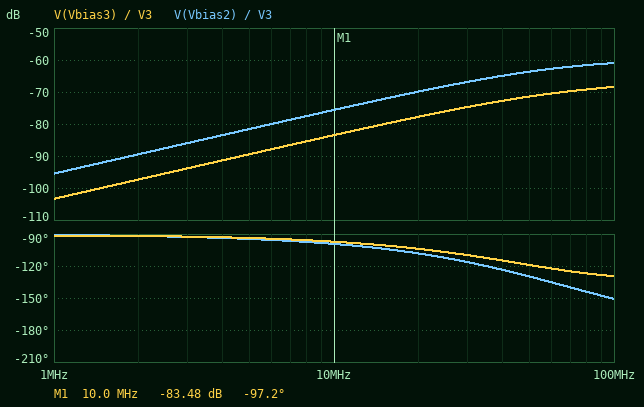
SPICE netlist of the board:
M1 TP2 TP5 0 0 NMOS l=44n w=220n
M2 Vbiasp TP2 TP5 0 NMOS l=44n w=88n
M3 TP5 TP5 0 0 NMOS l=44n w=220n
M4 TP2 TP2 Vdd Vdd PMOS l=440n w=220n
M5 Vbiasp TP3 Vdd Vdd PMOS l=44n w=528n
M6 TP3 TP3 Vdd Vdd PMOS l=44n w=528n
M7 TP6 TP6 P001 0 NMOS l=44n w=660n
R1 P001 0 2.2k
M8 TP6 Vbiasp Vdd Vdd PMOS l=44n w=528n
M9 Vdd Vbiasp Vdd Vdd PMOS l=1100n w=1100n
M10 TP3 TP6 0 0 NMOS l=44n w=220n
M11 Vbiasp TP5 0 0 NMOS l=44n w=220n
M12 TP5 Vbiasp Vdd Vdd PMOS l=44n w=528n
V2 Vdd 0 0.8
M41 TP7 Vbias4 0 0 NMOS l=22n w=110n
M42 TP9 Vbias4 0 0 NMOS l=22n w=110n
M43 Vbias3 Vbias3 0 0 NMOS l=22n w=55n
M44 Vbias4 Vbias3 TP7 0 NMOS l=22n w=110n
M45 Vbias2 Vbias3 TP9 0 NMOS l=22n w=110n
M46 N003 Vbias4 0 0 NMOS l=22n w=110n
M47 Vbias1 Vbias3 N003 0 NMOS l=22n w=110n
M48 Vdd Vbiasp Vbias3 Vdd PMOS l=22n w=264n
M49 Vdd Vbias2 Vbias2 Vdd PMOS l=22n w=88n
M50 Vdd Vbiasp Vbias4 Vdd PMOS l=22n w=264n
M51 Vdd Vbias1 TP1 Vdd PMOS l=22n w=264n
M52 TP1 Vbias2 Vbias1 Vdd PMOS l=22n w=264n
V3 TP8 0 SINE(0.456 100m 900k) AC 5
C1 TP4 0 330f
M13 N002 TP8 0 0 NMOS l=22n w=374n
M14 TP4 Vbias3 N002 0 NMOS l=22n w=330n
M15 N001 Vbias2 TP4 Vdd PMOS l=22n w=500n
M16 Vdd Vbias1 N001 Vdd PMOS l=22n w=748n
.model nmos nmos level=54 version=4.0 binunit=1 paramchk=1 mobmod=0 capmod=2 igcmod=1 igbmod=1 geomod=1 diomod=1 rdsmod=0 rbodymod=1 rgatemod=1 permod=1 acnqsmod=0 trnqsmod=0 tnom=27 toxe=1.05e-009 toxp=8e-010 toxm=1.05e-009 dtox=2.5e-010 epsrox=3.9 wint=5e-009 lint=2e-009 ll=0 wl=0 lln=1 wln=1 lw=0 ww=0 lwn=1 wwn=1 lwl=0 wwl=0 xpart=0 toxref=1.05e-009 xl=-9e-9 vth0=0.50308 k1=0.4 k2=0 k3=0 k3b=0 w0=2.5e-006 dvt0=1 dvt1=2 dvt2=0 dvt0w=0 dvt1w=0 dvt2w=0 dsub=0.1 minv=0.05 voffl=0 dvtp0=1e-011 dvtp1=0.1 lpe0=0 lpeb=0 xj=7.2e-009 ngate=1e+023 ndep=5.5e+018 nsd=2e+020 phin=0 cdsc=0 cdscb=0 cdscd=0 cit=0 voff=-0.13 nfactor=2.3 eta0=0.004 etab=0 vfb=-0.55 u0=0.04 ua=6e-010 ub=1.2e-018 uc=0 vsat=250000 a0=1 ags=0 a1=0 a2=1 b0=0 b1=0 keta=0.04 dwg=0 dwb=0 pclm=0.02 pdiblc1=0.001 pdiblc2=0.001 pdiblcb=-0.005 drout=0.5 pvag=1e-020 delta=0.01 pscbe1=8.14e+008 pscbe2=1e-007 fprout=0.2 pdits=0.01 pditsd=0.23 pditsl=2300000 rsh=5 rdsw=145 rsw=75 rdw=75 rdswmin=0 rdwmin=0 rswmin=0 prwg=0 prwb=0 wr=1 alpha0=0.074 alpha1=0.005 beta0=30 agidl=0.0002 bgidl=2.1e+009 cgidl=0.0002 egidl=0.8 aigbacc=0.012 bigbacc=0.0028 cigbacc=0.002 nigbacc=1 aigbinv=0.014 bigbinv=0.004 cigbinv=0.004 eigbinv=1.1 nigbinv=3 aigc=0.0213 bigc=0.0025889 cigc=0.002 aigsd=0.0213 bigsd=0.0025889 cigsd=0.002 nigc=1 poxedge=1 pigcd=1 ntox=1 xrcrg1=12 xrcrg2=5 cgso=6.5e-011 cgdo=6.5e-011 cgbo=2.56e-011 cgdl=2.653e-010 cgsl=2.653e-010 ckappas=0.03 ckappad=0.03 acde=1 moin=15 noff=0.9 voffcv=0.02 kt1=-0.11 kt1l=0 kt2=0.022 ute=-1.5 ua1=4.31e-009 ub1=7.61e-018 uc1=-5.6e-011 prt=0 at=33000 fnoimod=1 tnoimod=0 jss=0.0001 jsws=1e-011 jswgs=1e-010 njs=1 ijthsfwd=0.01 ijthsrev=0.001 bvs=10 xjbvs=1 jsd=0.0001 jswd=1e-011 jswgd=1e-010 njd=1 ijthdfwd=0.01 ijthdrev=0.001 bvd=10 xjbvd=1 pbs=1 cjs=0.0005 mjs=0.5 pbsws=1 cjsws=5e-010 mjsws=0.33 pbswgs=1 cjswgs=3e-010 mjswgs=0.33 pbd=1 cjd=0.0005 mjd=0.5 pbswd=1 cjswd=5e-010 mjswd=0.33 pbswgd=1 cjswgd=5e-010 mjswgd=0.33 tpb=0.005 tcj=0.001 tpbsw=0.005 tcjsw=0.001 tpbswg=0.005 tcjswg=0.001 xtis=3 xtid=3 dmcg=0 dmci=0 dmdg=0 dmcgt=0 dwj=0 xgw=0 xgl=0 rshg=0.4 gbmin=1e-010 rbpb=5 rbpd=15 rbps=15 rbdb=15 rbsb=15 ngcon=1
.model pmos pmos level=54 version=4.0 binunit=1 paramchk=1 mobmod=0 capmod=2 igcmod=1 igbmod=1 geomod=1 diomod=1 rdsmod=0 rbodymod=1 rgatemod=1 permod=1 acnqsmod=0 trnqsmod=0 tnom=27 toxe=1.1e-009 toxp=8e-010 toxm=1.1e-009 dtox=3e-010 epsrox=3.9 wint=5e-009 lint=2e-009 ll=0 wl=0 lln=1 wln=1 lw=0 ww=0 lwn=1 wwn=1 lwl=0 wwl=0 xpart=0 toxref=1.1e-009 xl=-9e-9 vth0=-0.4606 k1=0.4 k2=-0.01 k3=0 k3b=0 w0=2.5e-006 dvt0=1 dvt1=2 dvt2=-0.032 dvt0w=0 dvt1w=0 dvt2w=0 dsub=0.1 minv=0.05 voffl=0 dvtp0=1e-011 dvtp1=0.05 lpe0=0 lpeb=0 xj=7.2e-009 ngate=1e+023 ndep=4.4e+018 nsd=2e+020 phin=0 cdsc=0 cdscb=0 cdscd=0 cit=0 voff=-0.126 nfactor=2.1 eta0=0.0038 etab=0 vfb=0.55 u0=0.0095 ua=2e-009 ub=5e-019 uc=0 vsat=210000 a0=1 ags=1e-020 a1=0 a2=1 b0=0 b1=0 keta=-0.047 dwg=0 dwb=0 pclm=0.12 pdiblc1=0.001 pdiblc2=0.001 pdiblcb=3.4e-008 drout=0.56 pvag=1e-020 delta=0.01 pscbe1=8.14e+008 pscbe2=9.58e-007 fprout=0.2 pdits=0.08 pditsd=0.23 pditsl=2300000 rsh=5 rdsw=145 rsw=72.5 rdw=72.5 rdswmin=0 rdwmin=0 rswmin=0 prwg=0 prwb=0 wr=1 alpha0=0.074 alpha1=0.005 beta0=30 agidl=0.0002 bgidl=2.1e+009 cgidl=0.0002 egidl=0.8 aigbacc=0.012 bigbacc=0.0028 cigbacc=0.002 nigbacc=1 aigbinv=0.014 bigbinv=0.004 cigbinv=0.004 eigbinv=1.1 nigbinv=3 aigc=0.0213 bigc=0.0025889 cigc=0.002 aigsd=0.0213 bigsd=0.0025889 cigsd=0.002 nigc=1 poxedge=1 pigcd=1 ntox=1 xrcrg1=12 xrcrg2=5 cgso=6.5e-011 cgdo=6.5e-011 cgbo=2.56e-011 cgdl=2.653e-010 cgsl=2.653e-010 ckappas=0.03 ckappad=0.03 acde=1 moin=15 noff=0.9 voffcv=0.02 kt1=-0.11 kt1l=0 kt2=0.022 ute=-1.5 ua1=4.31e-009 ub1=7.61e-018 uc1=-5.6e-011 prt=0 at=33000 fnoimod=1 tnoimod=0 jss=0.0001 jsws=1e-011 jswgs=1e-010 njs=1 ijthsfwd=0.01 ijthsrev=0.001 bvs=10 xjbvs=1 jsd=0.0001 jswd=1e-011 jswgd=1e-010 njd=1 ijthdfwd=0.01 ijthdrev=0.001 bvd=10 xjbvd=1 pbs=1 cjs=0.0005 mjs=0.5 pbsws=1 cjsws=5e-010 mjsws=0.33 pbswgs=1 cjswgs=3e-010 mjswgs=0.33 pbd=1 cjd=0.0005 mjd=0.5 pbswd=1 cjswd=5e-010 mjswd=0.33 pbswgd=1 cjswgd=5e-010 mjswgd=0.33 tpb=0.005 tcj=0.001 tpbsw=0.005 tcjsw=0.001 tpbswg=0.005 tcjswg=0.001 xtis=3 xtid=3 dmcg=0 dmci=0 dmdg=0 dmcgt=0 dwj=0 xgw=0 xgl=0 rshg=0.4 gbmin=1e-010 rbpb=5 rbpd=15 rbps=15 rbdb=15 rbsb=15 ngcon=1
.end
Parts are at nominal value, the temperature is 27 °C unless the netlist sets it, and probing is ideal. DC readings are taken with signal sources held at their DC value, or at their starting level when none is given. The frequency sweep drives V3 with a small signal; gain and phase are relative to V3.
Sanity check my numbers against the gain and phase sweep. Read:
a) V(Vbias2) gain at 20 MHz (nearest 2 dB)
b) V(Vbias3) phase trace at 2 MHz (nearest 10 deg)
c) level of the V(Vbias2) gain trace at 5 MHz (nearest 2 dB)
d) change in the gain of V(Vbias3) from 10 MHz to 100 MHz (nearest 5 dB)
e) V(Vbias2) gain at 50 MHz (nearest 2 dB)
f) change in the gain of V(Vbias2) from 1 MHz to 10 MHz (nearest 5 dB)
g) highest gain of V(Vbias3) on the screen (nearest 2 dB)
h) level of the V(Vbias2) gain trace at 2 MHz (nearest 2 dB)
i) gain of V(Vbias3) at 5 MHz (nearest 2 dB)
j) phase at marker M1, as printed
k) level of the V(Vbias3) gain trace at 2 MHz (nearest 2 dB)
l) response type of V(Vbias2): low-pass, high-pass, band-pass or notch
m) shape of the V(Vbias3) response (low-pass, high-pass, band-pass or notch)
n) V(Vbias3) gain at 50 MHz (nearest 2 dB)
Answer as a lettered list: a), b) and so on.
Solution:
a) -70 dB
b) -90 deg
c) -82 dB
d) 15 dB
e) -64 dB
f) 20 dB
g) -68 dB
h) -90 dB
i) -90 dB
j) -97.2 deg
k) -98 dB
l) high-pass
m) high-pass
n) -72 dB
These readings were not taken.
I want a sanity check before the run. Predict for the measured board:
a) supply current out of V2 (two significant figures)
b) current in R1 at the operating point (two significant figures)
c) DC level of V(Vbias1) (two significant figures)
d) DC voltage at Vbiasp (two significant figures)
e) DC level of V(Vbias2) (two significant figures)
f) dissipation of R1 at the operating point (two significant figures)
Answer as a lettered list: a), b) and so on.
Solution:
a) 280 µA
b) 29 µA
c) 210 mV
d) 130 mV
e) 230 mV
f) 1.8 µW
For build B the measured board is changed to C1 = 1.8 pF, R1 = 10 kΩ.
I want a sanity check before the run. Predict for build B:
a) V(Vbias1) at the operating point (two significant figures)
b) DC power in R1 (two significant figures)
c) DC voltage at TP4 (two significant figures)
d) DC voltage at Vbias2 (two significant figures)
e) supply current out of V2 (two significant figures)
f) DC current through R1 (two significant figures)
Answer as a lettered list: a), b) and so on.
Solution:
a) 270 mV
b) 220 nW
c) 520 mV
d) 300 mV
e) 120 µA
f) 4.7 µA
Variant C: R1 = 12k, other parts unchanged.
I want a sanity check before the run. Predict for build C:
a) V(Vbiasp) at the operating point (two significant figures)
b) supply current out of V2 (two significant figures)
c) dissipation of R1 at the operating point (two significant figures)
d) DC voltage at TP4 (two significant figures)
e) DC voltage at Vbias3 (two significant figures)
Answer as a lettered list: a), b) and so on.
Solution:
a) 310 mV
b) 110 µA
c) 180 nW
d) 500 mV
e) 550 mV
